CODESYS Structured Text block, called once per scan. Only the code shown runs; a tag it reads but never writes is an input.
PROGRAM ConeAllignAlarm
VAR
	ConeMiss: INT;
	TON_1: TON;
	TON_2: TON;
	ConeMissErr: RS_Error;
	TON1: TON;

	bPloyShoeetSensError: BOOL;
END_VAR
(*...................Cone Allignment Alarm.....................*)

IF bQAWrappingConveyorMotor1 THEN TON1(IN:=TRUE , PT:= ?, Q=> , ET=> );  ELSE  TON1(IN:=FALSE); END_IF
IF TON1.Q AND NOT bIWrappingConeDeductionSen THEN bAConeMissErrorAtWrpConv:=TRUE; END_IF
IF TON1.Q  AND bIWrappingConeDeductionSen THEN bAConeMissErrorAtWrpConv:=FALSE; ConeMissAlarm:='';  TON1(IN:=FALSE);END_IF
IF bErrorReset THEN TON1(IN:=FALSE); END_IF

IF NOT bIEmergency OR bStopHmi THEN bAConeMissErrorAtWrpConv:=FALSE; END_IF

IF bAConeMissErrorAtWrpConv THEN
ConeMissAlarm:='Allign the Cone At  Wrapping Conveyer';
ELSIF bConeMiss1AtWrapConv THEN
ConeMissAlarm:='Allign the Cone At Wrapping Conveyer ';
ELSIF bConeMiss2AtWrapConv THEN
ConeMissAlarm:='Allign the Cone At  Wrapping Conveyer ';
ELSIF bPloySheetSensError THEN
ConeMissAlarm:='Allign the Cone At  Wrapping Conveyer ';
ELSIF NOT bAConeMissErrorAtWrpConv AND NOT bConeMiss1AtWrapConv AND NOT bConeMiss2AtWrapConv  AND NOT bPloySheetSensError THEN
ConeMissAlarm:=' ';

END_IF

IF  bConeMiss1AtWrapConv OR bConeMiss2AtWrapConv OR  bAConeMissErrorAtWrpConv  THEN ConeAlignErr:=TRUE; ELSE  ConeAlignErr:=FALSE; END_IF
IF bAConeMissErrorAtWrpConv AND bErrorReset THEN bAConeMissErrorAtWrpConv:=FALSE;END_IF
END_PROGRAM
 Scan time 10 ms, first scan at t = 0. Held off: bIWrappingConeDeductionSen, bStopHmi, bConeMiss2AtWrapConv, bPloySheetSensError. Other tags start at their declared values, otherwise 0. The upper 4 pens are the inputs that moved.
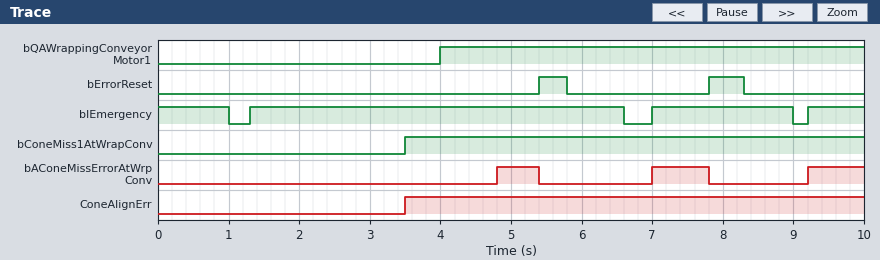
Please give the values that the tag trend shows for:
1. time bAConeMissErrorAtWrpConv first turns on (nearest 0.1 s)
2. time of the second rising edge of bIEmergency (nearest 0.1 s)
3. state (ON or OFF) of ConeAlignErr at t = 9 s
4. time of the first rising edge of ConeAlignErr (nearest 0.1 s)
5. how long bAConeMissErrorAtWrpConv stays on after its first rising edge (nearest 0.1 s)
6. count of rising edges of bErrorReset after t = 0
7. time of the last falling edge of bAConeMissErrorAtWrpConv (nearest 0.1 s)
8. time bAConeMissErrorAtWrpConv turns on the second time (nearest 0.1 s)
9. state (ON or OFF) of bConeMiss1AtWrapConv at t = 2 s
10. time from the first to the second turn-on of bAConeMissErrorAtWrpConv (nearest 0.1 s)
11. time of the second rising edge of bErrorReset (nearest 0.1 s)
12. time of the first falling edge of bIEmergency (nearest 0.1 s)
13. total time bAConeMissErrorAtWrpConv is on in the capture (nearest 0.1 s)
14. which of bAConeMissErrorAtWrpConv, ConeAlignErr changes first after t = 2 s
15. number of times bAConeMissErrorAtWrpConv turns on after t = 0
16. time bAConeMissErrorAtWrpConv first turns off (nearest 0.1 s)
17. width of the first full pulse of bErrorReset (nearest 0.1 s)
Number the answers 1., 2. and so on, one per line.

1. 4.8 s
2. 7.0 s
3. ON
4. 3.5 s
5. 0.6 s
6. 2
7. 7.8 s
8. 7.0 s
9. OFF
10. 2.2 s
11. 7.8 s
12. 1.0 s
13. 2.2 s
14. ConeAlignErr
15. 3
16. 5.4 s
17. 0.4 s
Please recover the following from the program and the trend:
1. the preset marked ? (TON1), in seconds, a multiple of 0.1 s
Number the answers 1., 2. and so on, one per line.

1. 0.8 s
